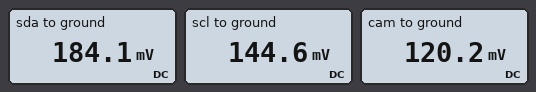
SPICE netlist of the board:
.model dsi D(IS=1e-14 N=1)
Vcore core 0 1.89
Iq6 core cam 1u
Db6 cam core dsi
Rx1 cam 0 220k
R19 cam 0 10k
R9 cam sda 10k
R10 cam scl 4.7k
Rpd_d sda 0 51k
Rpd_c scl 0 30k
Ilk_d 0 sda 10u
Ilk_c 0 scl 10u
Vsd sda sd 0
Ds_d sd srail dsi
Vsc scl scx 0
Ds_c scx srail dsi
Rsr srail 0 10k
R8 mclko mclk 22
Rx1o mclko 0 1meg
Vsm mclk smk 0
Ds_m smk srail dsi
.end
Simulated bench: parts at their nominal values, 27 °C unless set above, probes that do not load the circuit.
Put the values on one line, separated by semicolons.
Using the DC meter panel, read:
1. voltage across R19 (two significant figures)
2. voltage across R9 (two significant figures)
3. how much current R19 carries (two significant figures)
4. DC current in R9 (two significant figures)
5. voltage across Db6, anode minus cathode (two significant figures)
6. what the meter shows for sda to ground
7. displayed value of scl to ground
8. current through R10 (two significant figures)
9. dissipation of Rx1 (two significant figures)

120 mV; 64 mV; 12 µA; 6.4 µA; -1.8 V; 184.1 mV; 144.6 mV; 5.2 µA; 66 nW
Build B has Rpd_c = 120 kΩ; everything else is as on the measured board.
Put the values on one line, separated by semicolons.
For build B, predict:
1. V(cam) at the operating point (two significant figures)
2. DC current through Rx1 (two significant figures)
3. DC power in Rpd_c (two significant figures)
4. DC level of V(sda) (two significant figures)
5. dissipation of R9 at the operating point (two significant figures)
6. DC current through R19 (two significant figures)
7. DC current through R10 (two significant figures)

150 mV; 670 nA; 290 nW; 210 mV; 350 nW; 15 µA; 8.4 µA
